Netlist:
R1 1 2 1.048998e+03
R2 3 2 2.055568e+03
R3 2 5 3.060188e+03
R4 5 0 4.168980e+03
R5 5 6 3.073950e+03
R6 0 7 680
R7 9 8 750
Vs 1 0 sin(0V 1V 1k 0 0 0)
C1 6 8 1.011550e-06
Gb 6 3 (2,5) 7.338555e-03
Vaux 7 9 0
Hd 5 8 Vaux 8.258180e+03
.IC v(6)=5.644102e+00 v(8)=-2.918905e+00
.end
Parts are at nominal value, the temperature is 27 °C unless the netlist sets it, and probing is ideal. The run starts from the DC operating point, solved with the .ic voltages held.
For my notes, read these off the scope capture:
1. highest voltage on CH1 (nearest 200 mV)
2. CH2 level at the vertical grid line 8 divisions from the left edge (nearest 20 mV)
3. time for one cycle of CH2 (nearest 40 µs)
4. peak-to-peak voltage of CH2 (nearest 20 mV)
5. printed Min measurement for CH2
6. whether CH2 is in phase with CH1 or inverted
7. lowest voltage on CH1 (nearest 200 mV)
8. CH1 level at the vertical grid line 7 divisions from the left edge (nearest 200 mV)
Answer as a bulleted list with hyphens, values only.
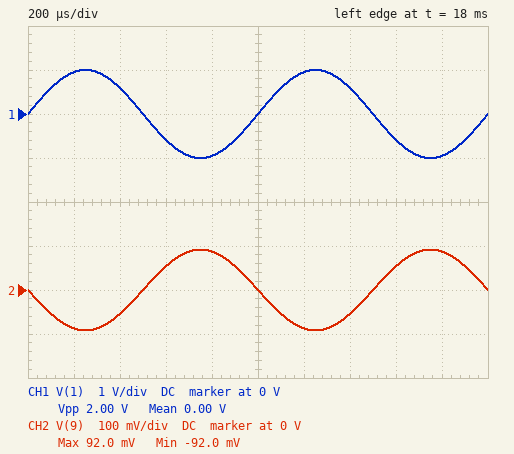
- 1.0 V
- 60 mV
- 1.00 ms
- 180 mV
- -92.0 mV
- inverted
- -1.0 V
- 600 mV
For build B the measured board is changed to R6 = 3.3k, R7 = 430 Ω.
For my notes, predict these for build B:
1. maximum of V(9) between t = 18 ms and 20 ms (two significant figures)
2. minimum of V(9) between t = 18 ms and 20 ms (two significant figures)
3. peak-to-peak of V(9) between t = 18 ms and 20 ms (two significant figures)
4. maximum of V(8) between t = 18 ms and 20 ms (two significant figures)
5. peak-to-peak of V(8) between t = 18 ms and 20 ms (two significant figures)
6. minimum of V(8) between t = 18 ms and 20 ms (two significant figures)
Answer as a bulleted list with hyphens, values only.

- 720 mV
- -720 mV
- 1.4 V
- 810 mV
- 1.6 V
- -810 mV
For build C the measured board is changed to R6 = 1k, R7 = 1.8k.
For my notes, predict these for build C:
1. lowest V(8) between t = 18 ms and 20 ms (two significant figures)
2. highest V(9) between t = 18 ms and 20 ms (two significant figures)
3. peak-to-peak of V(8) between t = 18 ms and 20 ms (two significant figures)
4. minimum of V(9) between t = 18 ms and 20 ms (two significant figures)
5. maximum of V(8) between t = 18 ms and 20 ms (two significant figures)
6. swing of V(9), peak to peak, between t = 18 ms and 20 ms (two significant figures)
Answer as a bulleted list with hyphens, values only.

- -490 mV
- 170 mV
- 980 mV
- -170 mV
- 490 mV
- 350 mV
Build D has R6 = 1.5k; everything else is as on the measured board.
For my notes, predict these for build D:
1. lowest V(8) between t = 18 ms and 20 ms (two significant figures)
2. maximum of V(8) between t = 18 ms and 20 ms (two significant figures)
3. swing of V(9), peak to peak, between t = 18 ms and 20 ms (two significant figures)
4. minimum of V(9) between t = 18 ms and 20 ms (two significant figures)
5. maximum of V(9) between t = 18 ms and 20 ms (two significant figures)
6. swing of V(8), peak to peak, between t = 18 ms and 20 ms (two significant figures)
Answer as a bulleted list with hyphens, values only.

- -350 mV
- 350 mV
- 470 mV
- -230 mV
- 230 mV
- 700 mV
